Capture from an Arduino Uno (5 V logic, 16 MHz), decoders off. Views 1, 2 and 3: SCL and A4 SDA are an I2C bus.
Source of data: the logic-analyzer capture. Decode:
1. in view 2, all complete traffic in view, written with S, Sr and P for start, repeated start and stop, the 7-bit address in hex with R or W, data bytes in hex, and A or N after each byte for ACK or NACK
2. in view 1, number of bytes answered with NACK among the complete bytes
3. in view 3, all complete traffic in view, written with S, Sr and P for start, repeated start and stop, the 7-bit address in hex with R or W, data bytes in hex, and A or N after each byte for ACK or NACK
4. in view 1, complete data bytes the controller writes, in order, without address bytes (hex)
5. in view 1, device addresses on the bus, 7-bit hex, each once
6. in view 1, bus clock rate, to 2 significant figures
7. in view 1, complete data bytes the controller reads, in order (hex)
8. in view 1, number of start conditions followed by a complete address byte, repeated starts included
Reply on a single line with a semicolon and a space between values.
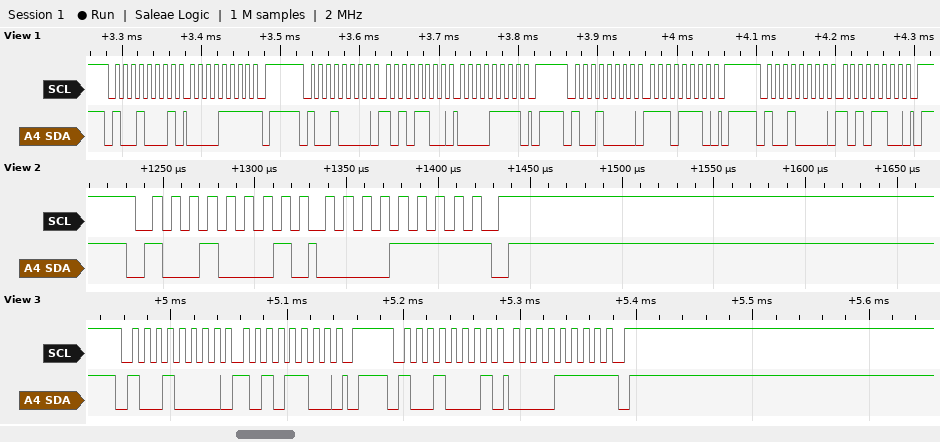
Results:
S 48R A 0F N P; 1; S 48W A AC A P S 48R A 0F N P; AC 0F EE AC; 0x48; 100 kHz; 0F; 4
